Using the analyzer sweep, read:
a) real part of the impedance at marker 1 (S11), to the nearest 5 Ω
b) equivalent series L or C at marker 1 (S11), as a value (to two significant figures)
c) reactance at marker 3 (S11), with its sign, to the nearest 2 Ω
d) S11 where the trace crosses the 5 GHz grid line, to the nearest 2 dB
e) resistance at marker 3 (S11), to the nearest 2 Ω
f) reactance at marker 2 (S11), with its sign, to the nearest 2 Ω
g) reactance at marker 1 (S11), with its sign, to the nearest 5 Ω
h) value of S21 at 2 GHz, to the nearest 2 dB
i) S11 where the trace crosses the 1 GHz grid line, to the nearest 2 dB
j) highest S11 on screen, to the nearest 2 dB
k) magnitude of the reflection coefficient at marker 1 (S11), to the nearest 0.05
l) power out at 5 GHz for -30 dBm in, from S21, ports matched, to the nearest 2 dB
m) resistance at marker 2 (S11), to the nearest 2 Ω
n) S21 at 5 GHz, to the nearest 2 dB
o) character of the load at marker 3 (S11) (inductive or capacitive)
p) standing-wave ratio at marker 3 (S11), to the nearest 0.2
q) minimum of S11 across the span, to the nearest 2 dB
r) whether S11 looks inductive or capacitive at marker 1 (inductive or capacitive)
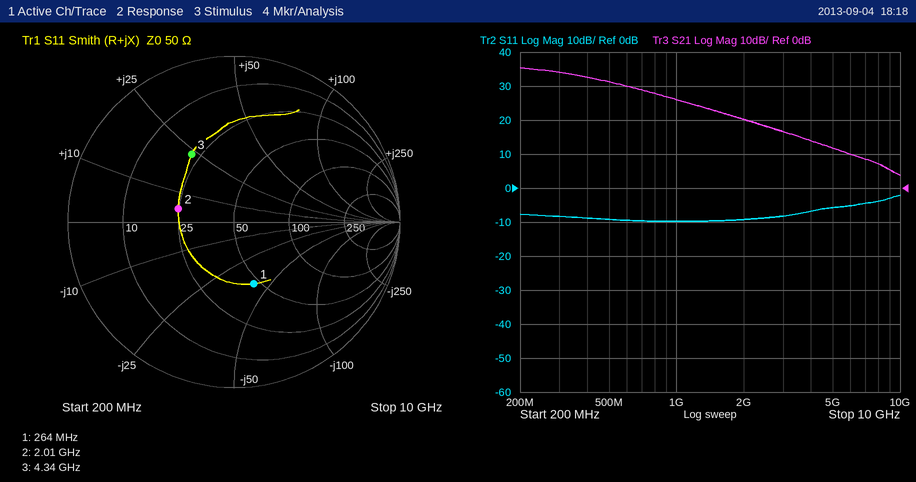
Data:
45 Ω
15 pF
+24 Ω
-6 dB
22 Ω
+4 Ω
-40 Ω
20 dB
-10 dB
-2 dB
0.40
-18 dBm
24 Ω
12 dB
inductive
2.8
-10 dB
capacitive
